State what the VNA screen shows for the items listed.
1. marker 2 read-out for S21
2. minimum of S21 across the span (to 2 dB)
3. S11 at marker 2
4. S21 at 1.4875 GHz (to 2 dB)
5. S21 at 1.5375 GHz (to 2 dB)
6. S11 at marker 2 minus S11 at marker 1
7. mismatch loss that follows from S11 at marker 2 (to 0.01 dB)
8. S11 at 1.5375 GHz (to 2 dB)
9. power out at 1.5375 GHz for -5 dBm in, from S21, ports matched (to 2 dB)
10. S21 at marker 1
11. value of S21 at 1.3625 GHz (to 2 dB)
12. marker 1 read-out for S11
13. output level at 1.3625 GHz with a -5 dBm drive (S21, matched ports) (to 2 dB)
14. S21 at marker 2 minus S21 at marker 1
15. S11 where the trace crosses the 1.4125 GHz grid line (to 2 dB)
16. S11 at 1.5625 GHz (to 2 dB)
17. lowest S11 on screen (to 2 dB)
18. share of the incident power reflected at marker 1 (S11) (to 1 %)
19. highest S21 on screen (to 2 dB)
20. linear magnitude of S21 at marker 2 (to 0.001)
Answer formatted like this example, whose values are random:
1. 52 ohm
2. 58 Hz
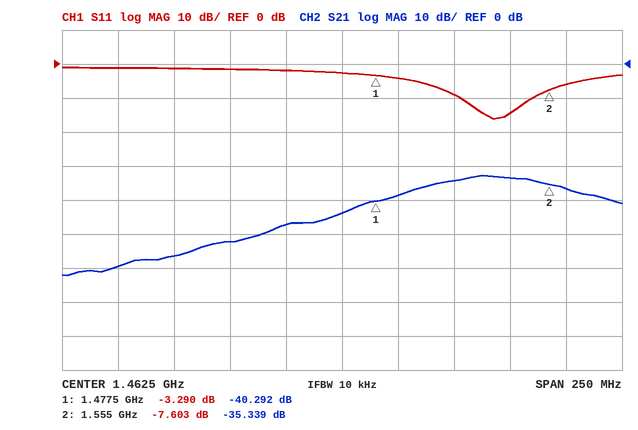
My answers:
1. -35.339 dB
2. -62 dB
3. -7.603 dB
4. -38 dB
5. -34 dB
6. -4.313 dB
7. 0.83 dB
8. -14 dB
9. -38 dBm
10. -40.292 dB
11. -60 dB
12. -3.290 dB
13. -64 dBm
14. 4.953 dB
15. -2 dB
16. -6 dB
17. -16 dB
18. 47 %
19. -32 dB
20. 0.017
